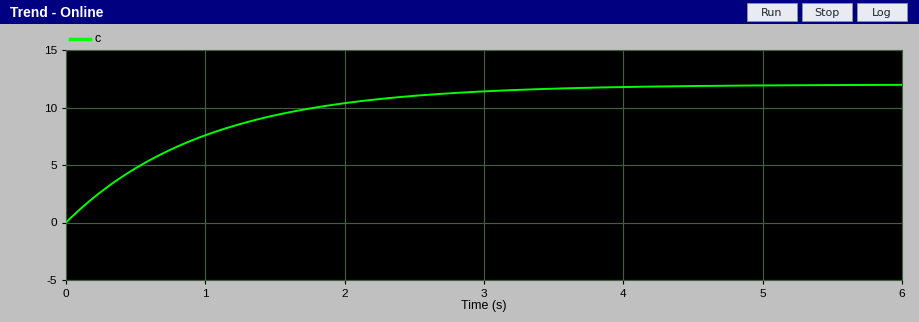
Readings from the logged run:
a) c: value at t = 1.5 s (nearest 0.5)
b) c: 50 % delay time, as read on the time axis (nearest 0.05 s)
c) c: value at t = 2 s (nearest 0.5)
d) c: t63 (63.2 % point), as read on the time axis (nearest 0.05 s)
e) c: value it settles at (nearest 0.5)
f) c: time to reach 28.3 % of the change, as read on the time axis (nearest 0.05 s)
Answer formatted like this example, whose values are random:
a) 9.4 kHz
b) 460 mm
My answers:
a) 9.5
b) 0.70 s
c) 10.5
d) 1.00 s
e) 12.0
f) 0.35 s
